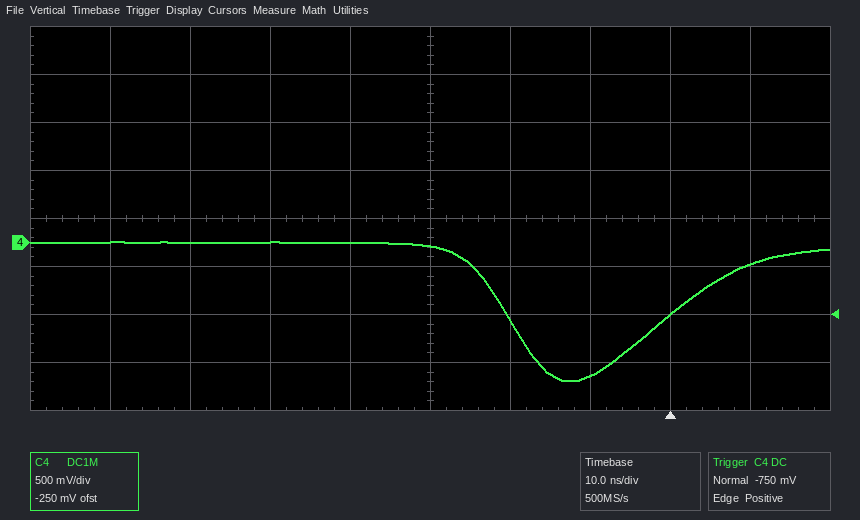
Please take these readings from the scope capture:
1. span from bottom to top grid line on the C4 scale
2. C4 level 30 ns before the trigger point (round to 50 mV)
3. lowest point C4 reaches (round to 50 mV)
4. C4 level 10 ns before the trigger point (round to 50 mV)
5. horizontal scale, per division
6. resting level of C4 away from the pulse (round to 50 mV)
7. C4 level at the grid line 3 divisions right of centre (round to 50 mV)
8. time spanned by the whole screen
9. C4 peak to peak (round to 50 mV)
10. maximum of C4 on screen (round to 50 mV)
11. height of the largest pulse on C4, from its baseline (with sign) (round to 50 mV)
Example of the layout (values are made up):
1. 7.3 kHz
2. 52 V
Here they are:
1. 4 V
2. -50 mV
3. -1.45 V
4. -1.40 V
5. 10 ns
6. 0 mV
7. -750 mV
8. 100 ns
9. 1.45 V
10. 0 mV
11. -1.45 V
